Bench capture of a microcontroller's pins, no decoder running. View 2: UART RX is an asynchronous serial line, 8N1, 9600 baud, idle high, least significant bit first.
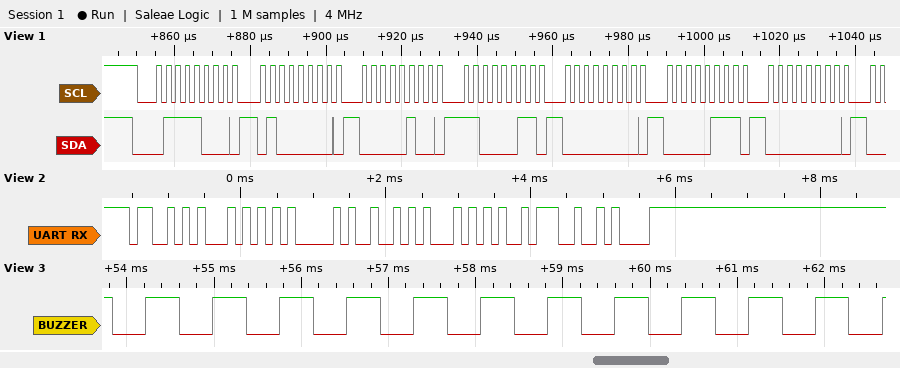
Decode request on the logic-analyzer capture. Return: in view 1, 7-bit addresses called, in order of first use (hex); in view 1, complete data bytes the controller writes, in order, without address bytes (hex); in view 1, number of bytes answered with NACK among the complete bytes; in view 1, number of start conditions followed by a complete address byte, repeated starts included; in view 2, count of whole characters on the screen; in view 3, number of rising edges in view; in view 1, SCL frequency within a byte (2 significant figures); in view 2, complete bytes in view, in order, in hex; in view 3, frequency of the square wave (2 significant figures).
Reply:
0x3C
40 04 C3 00 07 00
0
1
7
12
400 kHz
53 54 41 52 54 3A 0A
1.3 kHz
